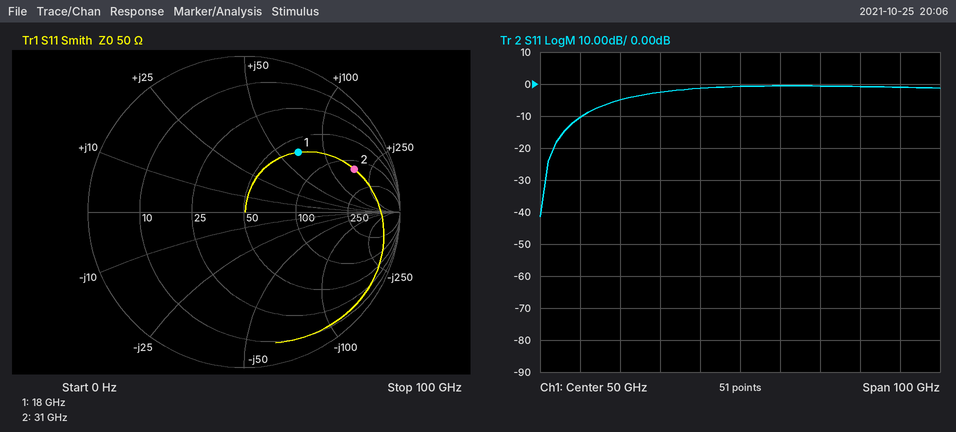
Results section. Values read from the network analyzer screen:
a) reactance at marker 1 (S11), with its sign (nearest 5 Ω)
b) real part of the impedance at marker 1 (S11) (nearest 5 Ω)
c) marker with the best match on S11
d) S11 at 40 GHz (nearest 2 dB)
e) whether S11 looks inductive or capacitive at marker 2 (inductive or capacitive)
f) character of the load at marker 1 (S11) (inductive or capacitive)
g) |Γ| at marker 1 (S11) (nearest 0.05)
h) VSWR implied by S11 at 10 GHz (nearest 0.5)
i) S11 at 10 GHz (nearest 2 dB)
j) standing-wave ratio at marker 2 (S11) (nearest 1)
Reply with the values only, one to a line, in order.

+65 Ω
65 Ω
marker 1
-2 dB
inductive
inductive
0.50
2.0
-10 dB
7
